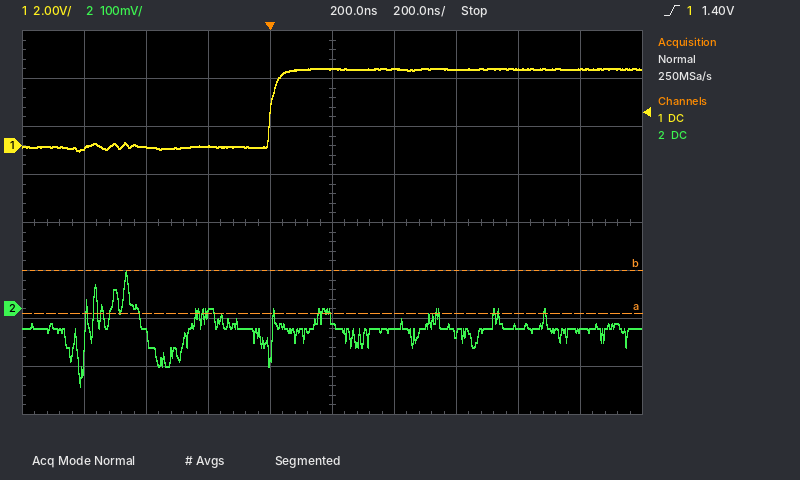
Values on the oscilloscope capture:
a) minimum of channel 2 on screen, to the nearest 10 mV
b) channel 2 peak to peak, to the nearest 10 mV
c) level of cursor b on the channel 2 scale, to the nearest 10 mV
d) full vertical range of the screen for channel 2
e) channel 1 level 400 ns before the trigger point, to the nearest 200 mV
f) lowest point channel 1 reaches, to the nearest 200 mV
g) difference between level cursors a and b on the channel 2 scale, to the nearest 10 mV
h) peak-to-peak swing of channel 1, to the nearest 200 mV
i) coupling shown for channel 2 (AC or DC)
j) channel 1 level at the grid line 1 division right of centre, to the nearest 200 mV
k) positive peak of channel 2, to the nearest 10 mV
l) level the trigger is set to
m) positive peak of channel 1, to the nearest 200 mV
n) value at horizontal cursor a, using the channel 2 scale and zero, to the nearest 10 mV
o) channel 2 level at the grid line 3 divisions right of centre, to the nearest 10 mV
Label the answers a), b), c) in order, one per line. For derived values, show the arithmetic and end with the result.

a) -160 mV
b) 80 mV − (-160 mV) = 240 mV
c) 80 mV
d) 800 mV
e) 0.0 V
f) -200 mV
g) 90 mV
h) 3.2 V − (-200 mV) = 3.4 V
i) DC
j) 3.2 V
k) 80 mV
l) 1.40 V
m) 3.2 V
n) -10 mV
o) -40 mV
